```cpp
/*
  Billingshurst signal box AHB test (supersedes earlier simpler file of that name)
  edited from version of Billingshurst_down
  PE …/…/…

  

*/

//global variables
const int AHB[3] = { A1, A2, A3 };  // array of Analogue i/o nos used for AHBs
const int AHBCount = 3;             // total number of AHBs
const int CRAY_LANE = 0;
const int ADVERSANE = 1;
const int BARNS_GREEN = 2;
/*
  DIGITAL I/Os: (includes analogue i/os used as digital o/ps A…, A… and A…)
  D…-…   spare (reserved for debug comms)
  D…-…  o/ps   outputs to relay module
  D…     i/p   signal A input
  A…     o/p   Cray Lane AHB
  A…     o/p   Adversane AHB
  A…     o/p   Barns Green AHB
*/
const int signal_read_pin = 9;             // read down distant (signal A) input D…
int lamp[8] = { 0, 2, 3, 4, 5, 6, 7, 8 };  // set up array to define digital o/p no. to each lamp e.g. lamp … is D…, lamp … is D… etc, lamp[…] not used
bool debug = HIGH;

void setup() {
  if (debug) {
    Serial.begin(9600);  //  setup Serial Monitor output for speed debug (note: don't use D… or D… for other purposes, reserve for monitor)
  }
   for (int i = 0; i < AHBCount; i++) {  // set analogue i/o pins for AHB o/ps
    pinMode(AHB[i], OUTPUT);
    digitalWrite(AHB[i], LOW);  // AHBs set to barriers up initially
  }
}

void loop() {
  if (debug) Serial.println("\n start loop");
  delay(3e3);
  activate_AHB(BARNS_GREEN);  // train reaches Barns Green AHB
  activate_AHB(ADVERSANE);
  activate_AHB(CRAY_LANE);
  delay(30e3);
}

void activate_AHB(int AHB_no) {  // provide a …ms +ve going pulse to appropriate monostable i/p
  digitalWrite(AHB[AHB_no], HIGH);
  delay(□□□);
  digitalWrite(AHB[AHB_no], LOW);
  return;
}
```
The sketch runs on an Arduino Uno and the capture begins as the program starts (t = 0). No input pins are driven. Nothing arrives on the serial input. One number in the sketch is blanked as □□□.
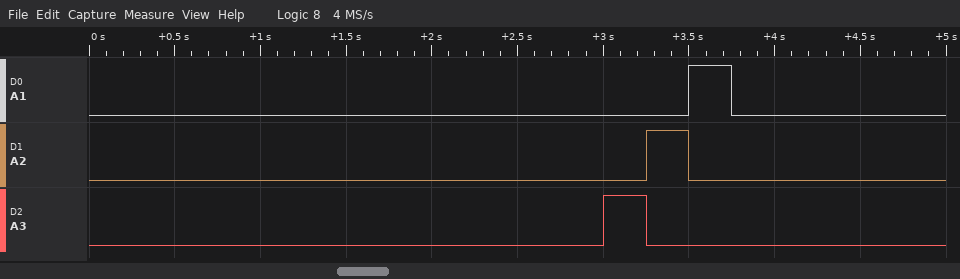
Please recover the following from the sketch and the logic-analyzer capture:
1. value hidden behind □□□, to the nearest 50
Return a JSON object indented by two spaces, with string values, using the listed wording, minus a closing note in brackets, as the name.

{
  "value hidden behind □□□, to the nearest 50": "250"
}
